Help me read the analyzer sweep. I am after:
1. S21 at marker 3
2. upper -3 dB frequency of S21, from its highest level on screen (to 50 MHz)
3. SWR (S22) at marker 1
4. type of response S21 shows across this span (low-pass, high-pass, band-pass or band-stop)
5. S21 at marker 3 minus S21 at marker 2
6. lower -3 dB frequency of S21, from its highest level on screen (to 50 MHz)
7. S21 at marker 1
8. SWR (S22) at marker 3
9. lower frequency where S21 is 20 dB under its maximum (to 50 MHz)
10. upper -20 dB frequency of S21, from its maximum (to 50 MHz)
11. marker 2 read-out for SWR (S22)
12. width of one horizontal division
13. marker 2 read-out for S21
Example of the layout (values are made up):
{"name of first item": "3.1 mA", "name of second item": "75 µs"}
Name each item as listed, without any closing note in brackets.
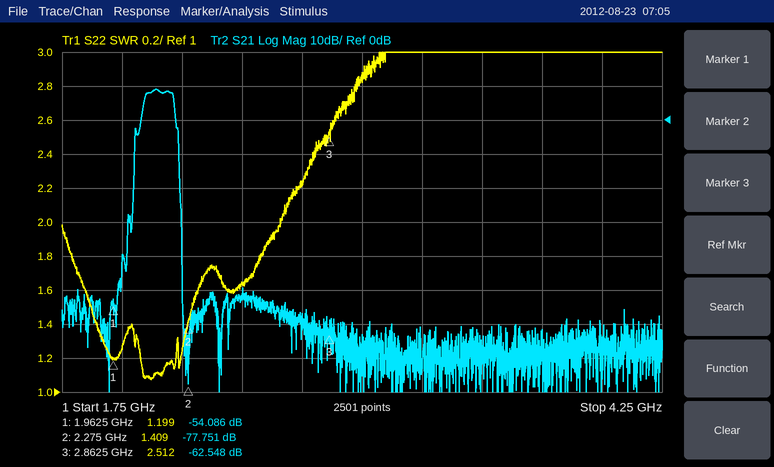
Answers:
{"S21 at marker 3": "-62.548 dB", "upper -3 dB frequency of S21, from its highest level on screen": "2.20 GHz", "SWR (S22) at marker 1": "1.199", "type of response S21 shows across this span": "band-pass", "S21 at marker 3 minus S21 at marker 2": "15.203 dB", "lower -3 dB frequency of S21, from its highest level on screen": "2.10 GHz", "S21 at marker 1": "-54.086 dB", "SWR (S22) at marker 3": "2.512", "lower frequency where S21 is 20 dB under its maximum": "2.05 GHz", "upper -20 dB frequency of S21, from its maximum": "2.25 GHz", "marker 2 read-out for SWR": "1.409", "width of one horizontal division": "250 MHz", "marker 2 read-out for S21": "-77.751 dB"}
